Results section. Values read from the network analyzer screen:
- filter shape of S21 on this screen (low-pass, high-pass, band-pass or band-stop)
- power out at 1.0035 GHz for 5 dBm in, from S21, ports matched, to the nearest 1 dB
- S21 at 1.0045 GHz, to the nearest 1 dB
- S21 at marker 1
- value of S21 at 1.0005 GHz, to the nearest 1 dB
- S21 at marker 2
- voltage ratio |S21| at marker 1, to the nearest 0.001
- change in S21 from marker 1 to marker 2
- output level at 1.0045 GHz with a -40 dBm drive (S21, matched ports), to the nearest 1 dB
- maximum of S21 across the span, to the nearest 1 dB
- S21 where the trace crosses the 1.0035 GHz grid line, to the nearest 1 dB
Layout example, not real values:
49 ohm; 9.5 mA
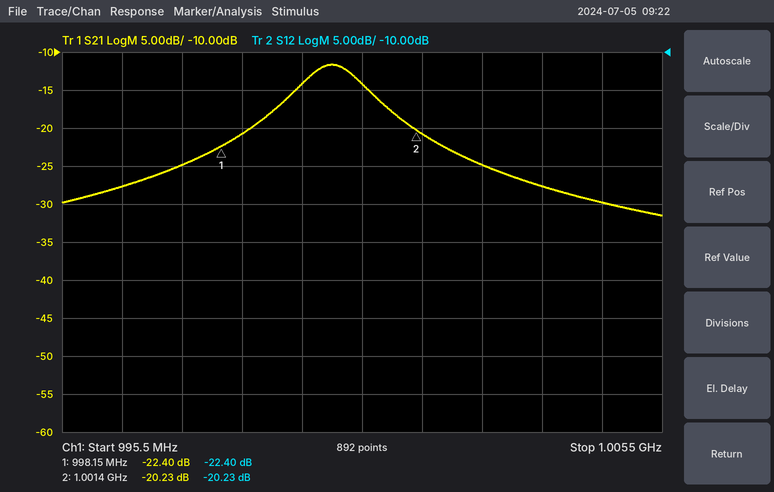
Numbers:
band-pass; -23 dBm; -30 dB; -22.40 dB; -14 dB; -20.23 dB; 0.076; 2.17 dB; -70 dBm; -12 dB; -28 dB
